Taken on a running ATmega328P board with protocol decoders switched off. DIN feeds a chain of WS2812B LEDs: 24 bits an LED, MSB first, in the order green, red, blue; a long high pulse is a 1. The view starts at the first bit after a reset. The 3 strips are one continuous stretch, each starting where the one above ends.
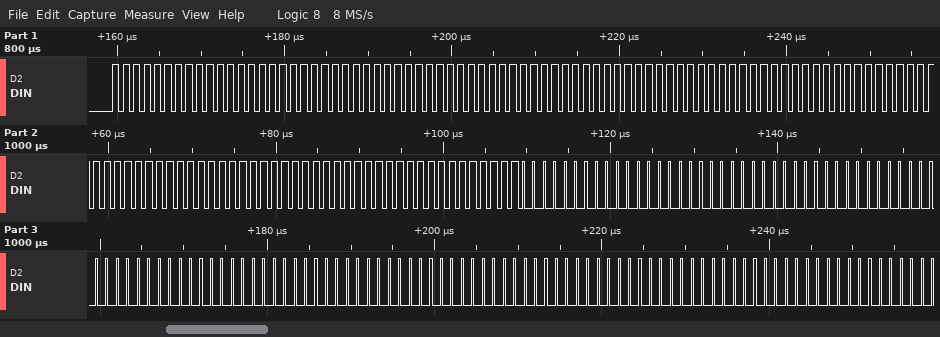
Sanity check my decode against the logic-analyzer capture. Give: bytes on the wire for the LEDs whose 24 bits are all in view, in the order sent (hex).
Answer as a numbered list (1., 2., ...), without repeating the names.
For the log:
1. FF FF FF FF FF FF FF FF FF FF FF FF FF FF FF 00 00 00 00 00 00 00 00 00 00 00 00 00 00 00
